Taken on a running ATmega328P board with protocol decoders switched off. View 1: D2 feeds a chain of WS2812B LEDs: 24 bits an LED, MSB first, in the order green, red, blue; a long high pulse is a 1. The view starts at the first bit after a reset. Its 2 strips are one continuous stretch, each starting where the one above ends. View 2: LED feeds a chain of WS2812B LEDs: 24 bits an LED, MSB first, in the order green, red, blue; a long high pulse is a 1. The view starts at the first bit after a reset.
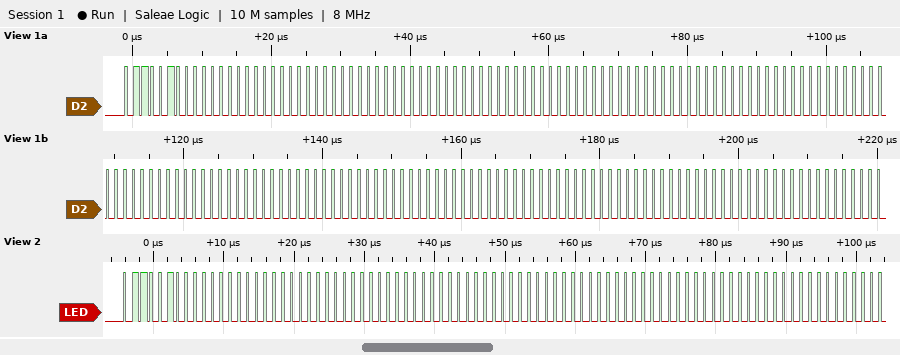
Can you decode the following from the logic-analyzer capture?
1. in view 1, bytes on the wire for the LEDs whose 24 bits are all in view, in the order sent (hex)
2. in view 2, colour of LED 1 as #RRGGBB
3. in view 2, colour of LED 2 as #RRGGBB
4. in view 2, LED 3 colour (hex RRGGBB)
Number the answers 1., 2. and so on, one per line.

1. 64 00 00 00 00 00 00 00 00 00 00 00 00 00 00 00 00 00 00 00 00
2. #006400
3. #000000
4. #000000
